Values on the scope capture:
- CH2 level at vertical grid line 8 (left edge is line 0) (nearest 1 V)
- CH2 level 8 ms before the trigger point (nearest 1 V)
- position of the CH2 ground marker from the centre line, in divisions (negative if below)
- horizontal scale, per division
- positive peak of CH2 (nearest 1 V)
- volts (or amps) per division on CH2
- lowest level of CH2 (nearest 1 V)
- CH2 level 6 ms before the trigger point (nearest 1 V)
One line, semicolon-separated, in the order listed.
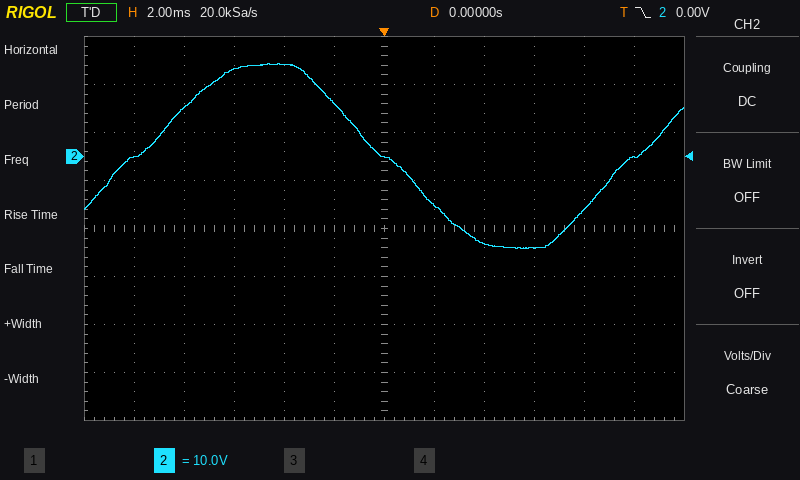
-18 V; 10 V; +1.5 div; 2 ms; 19 V; 10 V; -19 V; 18 V
